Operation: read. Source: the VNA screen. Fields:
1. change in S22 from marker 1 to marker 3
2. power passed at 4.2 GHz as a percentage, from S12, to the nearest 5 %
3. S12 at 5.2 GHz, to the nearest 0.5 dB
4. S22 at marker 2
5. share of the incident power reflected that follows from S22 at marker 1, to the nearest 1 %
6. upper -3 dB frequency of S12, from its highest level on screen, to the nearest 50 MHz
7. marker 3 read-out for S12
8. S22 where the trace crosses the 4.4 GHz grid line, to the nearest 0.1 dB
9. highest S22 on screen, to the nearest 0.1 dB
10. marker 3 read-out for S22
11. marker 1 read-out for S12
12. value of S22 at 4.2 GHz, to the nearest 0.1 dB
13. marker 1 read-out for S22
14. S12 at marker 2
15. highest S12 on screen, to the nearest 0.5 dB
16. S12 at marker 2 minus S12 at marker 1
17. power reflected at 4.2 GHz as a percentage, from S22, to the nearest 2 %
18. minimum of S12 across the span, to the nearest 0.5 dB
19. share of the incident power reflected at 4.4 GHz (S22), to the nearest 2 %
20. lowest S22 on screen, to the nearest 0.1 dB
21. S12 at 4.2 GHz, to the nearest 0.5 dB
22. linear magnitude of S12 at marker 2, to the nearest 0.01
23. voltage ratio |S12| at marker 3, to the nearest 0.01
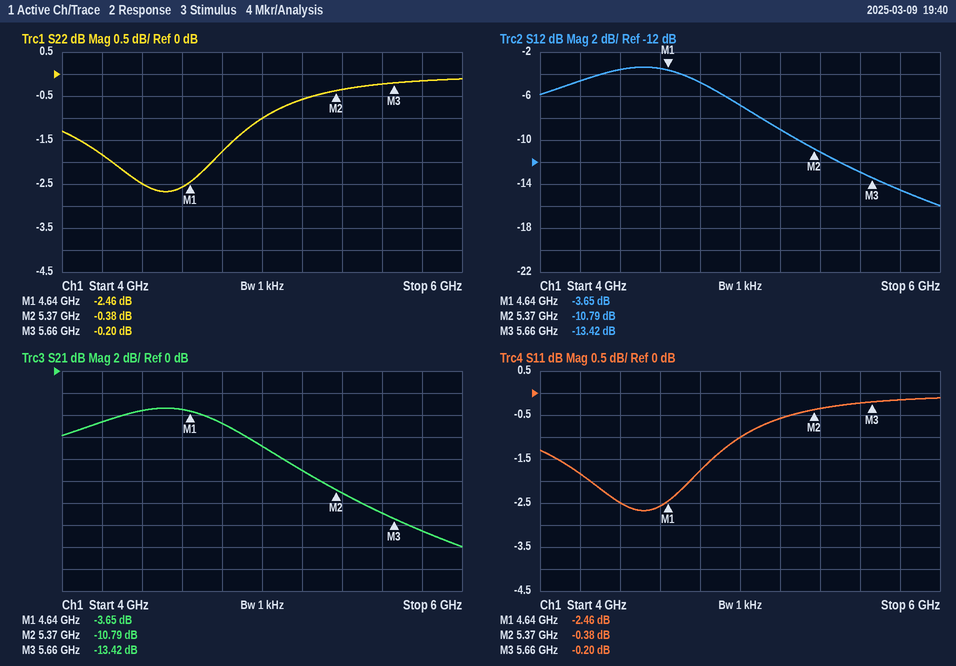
2.26 dB
35 %
-9.0 dB
-0.38 dB
57 %
4.95 GHz
-13.42 dB
-2.5 dB
-0.1 dB
-0.20 dB
-3.65 dB
-1.8 dB
-2.46 dB
-10.79 dB
-3.5 dB
-7.14 dB
66 %
-16.0 dB
56 %
-2.7 dB
-4.5 dB
0.29
0.21
